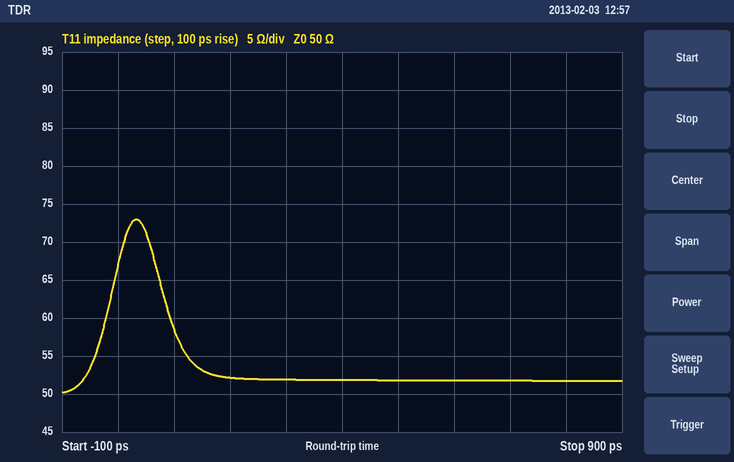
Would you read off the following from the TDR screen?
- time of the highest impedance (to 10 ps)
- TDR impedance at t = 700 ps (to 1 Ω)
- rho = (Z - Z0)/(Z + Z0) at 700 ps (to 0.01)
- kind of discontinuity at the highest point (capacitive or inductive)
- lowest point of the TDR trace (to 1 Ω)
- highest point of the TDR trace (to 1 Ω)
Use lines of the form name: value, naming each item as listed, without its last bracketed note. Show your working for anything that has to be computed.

time of the highest impedance: 30 ps
TDR impedance at t = 700 ps: 52 Ω
rho = (Z - Z0)/(Z + Z0) at 700 ps: (52 − 50)/(52 + 50) ≈ +0.02
kind of discontinuity at the highest point: inductive
lowest point of the TDR trace: 50 Ω
highest point of the TDR trace: 73 Ω
